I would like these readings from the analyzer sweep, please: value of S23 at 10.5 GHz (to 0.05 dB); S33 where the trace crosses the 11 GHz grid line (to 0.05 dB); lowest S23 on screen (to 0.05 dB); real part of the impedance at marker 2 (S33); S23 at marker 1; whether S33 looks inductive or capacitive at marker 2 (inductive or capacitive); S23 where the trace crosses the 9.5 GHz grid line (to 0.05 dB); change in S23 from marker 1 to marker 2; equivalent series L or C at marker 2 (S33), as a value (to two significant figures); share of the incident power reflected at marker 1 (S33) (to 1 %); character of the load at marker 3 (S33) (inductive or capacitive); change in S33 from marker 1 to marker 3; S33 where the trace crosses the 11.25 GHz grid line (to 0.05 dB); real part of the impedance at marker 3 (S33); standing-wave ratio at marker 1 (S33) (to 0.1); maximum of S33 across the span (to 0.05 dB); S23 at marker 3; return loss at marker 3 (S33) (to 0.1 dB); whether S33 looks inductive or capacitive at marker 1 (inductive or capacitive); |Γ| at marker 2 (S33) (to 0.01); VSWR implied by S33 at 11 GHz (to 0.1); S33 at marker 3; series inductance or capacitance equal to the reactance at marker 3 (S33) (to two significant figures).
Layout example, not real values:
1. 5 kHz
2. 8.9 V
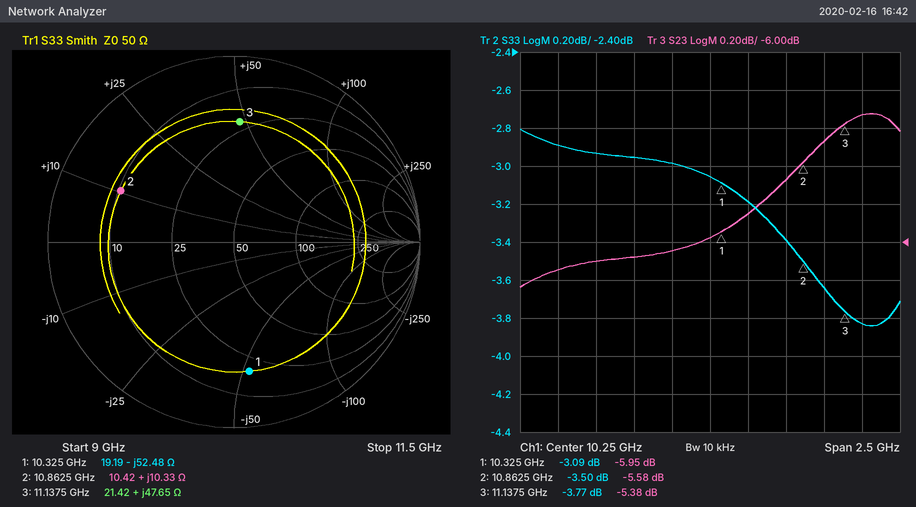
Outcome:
1. -5.85 dB
2. -3.65 dB
3. -6.25 dB
4. 10.42 Ω
5. -5.95 dB
6. inductive
7. -6.10 dB
8. 0.37 dB
9. 150 pH
10. 49 %
11. inductive
12. -0.68 dB
13. -3.85 dB
14. 21.42 Ω
15. 5.7
16. -2.80 dB
17. -5.38 dB
18. 3.8 dB
19. capacitive
20. 0.67
21. 4.8
22. -3.77 dB
23. 680 pH
